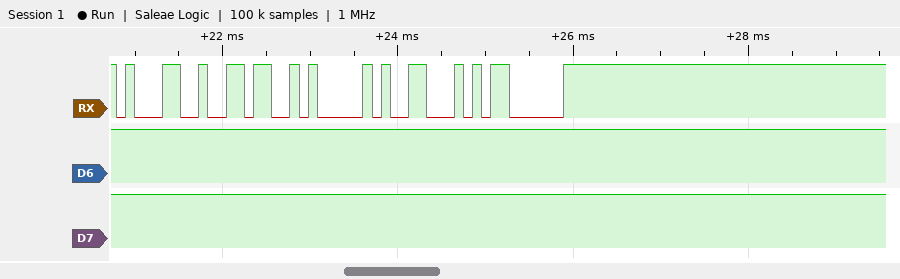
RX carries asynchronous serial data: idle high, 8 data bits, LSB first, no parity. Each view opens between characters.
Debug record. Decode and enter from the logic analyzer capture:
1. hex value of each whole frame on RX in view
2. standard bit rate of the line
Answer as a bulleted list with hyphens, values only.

- 31, 36, 41, 46, 03
- 9600 baud
